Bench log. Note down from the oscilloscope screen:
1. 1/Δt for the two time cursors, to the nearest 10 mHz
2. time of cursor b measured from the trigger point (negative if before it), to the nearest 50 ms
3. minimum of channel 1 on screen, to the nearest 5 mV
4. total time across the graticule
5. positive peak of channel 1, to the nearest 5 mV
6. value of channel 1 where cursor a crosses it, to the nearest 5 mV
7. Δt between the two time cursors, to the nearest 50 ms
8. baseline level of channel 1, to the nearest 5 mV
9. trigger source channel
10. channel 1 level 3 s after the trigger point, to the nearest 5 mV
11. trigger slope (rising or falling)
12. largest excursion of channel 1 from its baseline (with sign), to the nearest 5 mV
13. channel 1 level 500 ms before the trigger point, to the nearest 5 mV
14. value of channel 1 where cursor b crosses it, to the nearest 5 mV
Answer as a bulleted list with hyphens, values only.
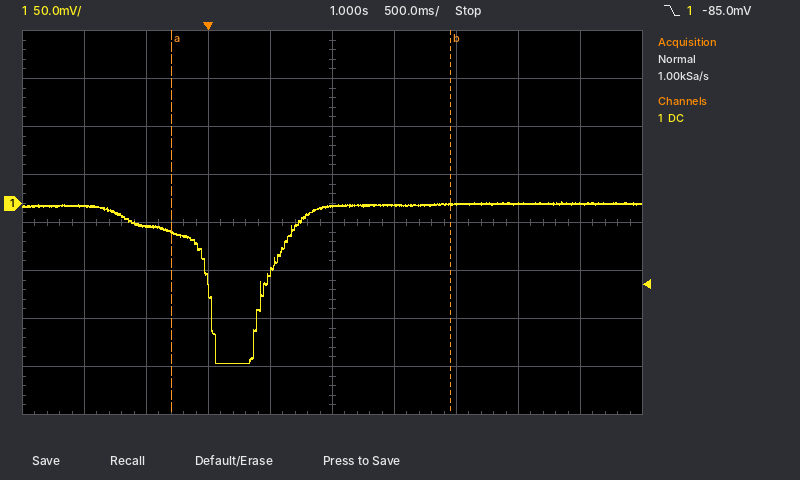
- 440 mHz
- +1.95 s
- -165 mV
- 5 s
- 0 mV
- -30 mV
- 2.25 s
- 0 mV
- channel 1
- 0 mV
- falling
- -165 mV
- -25 mV
- 0 mV
